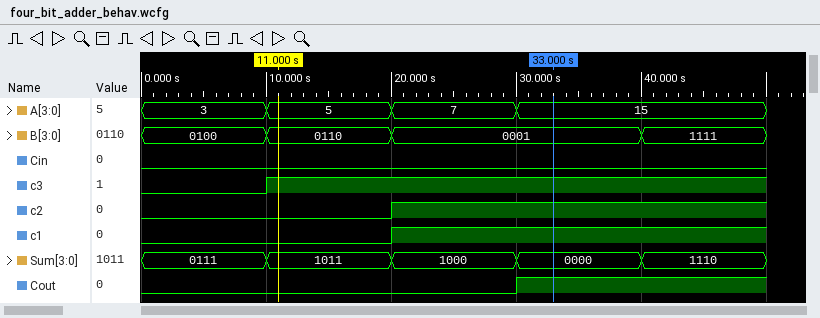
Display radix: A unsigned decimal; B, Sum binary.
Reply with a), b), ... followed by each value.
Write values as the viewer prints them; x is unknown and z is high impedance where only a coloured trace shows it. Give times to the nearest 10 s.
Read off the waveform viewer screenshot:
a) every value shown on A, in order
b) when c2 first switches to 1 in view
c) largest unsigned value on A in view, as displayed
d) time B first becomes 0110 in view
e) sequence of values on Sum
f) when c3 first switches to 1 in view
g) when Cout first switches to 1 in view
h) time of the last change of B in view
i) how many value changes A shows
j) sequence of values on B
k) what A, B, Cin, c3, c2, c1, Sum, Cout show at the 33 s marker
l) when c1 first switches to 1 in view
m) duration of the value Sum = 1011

a) 3, 5, 7, 15
b) 20 s
c) 15
d) 10 s
e) 0111, 1011, 1000, 0000, 1110
f) 10 s
g) 30 s
h) 40 s
i) 3
j) 0100, 0110, 0001, 1111
k) A=15, B=0001, Cin=0, c3=1, c2=1, c1=1, Sum=0000, Cout=1
l) 20 s
m) 10 s
